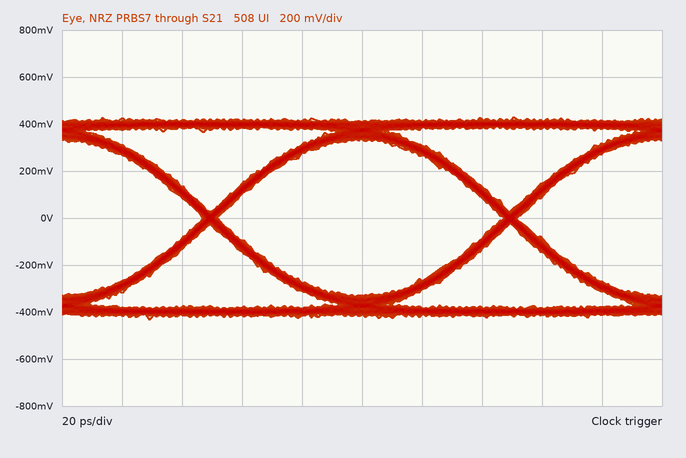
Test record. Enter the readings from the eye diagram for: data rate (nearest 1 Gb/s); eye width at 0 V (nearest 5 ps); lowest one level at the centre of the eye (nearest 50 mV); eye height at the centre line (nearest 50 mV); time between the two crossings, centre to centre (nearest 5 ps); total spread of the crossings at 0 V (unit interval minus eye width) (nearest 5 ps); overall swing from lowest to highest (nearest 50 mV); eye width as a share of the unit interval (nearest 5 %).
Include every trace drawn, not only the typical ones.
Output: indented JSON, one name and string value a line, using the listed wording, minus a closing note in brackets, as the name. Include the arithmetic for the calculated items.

{
  "data rate": "10 Gb/s",
  "eye width at 0 V": "95 ps",
  "lowest one level at the centre of the eye": "350 mV",
  "eye height at the centre line": "650 mV",
  "time between the two crossings, centre to centre": "100 ps",
  "total spread of the crossings at 0 V (unit interval minus eye width)": "5 ps",
  "overall swing from lowest to highest": "850 mV",
  "eye width as a share of the unit interval": "95 ps / 100 ps ≈ 95 %"
}
